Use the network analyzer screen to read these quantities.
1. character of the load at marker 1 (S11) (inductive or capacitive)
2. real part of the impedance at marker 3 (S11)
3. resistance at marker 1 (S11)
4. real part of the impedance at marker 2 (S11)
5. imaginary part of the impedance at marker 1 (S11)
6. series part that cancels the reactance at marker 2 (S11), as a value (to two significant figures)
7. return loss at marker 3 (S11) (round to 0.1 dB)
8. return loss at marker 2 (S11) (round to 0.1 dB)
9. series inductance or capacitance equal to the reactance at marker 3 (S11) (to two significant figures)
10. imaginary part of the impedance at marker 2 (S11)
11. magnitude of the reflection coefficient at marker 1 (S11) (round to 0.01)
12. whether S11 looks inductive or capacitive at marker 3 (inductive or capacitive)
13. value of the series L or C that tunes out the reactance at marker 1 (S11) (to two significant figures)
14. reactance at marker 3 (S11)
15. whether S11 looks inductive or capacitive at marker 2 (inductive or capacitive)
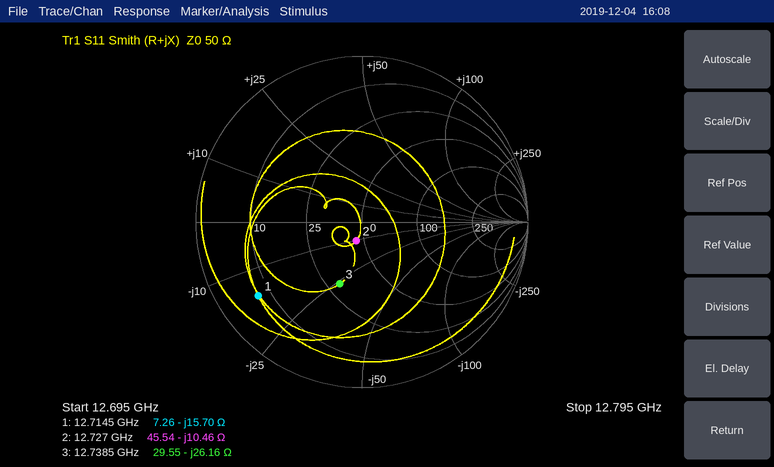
capacitive
29.55 Ω
7.26 Ω
45.54 Ω
-15.70 Ω
130 pH
8.0 dB
18.5 dB
480 fF
-10.46 Ω
0.77
capacitive
200 pH
-26.16 Ω
capacitive
